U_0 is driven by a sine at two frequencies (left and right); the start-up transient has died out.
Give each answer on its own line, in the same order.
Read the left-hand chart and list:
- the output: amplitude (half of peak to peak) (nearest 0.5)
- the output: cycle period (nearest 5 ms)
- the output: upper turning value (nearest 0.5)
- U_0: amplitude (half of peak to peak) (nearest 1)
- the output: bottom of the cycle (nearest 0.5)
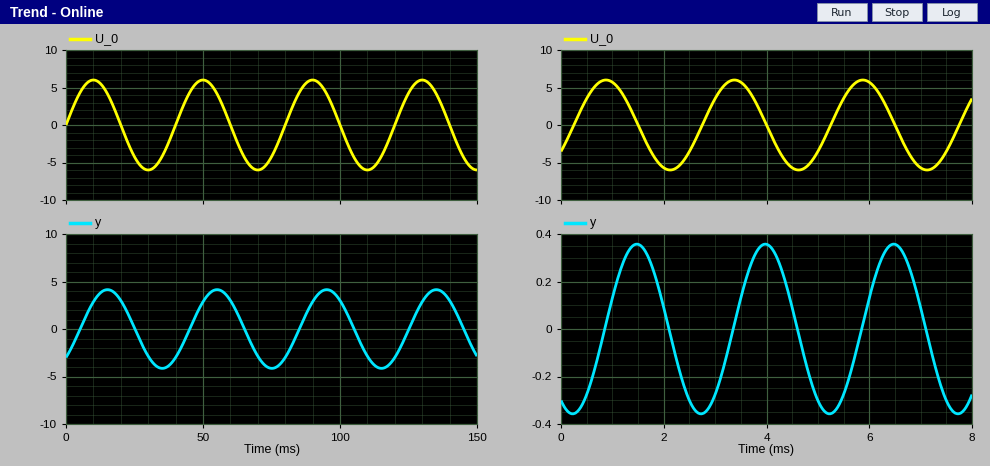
4.0
40 ms
4.0
6
-4.0
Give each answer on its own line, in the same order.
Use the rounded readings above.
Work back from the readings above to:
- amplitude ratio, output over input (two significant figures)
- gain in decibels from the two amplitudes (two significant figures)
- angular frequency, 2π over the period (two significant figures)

0.67
-3.5 dB
0.16 rad/ms
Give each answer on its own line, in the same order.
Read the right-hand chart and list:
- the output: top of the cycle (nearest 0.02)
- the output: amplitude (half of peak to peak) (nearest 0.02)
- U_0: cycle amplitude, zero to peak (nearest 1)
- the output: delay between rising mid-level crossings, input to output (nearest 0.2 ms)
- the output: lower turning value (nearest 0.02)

0.36
0.36
6
0.6 ms
-0.36
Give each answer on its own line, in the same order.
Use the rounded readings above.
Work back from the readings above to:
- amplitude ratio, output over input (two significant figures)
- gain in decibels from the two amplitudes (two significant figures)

0.060
-24 dB
